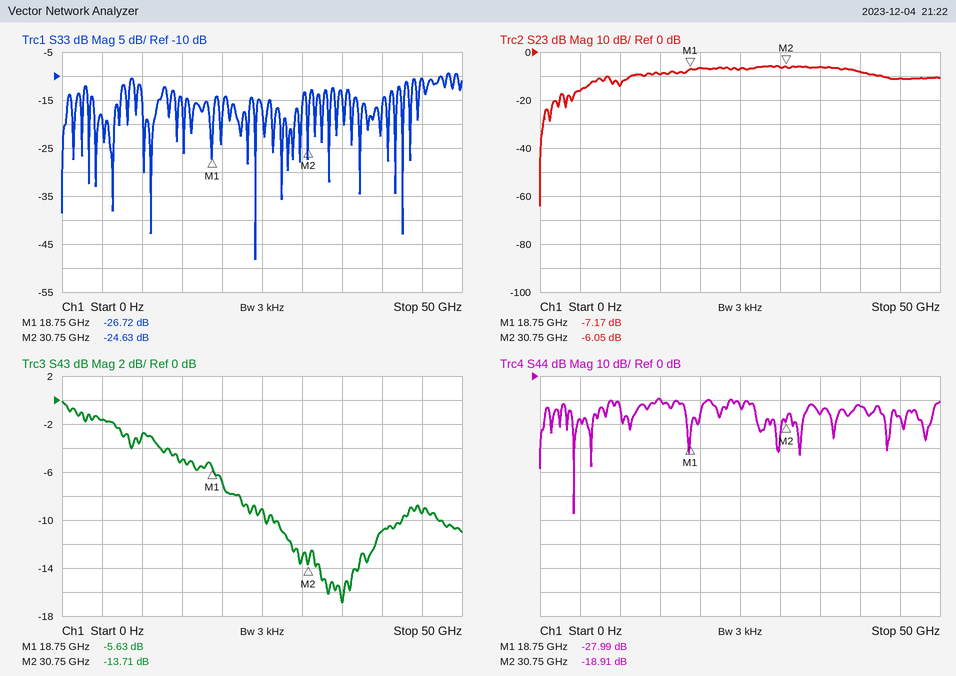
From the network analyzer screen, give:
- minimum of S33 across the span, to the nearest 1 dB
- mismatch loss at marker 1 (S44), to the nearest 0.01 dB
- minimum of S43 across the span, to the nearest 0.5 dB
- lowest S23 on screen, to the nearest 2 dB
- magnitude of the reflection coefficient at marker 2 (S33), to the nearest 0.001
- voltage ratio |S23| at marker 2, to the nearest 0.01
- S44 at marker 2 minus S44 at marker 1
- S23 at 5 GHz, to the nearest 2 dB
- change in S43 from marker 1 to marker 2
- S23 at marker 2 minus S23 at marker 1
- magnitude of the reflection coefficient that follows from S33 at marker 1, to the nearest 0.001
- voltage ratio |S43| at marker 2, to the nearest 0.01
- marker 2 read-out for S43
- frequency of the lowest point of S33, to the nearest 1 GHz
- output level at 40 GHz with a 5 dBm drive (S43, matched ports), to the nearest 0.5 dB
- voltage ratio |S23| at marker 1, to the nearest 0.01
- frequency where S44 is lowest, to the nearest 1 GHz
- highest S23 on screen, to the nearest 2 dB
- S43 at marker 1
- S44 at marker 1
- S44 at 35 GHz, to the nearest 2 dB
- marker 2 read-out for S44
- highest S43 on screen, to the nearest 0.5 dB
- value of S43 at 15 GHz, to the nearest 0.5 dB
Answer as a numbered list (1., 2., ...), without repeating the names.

1. -48 dB
2. 0.01 dB
3. -17.0 dB
4. -64 dB
5. 0.059
6. 0.50
7. 9.08 dB
8. -16 dB
9. -8.08 dB
10. 1.12 dB
11. 0.046
12. 0.21
13. -13.71 dB
14. 24 GHz
15. -6.0 dBm
16. 0.44
17. 4 GHz
18. -6 dB
19. -5.63 dB
20. -27.99 dB
21. -16 dB
22. -18.91 dB
23. 0.0 dB
24. -5.0 dB
